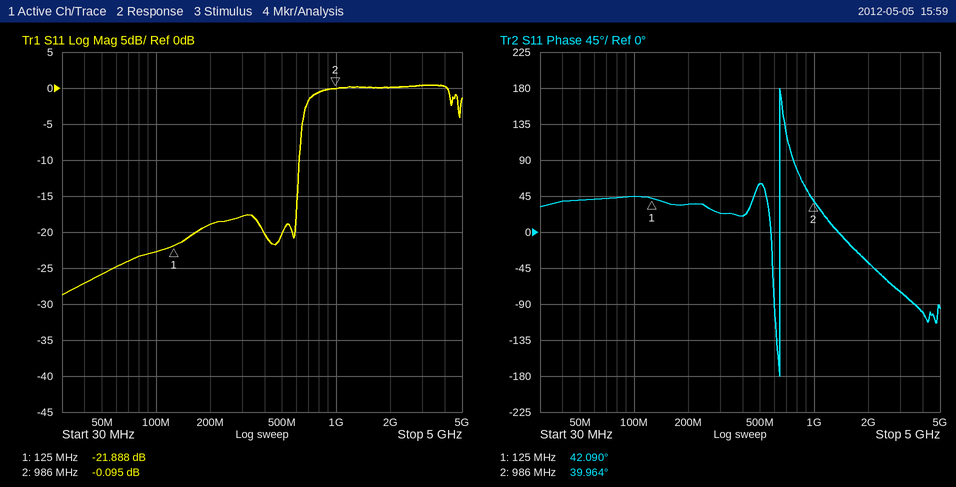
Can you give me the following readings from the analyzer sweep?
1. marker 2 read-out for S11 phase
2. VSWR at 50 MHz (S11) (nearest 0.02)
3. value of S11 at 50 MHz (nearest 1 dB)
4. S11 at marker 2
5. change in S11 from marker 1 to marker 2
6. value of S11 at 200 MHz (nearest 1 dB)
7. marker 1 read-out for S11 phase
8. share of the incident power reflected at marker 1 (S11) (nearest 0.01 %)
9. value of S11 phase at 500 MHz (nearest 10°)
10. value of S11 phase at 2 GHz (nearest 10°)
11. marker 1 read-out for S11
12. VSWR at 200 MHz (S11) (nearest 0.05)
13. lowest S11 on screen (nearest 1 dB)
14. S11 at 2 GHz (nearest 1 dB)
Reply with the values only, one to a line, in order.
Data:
39.964°
1.10
-26 dB
-0.095 dB
21.793 dB
-19 dB
42.090°
0.65 %
60°
-40°
-21.888 dB
1.25
-29 dB
0 dB
